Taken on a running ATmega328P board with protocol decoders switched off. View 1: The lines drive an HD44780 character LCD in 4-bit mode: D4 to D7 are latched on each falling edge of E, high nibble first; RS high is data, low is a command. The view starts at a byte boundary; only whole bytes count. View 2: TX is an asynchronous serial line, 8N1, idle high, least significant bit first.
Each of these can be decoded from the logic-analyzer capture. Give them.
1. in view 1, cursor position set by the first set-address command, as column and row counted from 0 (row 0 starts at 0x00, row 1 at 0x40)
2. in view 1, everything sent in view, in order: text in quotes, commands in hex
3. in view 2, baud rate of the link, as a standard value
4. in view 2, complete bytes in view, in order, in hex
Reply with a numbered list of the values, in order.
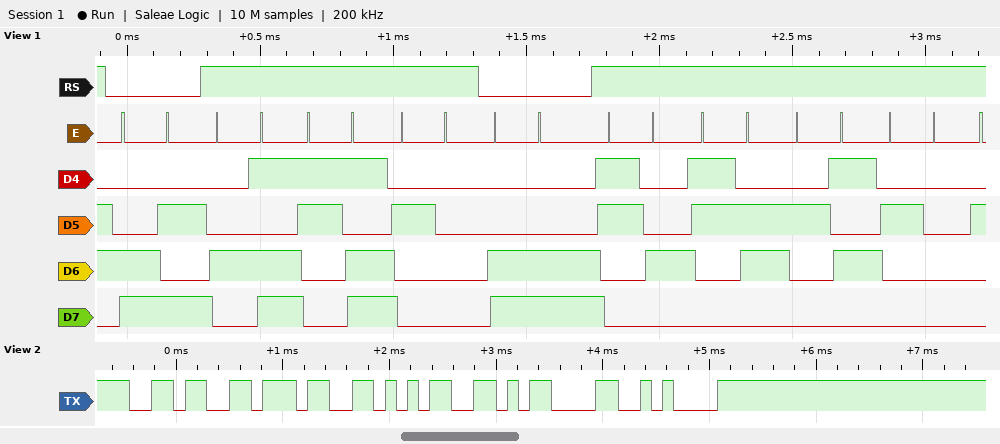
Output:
1. column 10, row 1
2. 0xCA "M= " 0xCC "46% "
3. 9600 baud
4. 0x36 0x37 0x35 0x0D 0x0A
